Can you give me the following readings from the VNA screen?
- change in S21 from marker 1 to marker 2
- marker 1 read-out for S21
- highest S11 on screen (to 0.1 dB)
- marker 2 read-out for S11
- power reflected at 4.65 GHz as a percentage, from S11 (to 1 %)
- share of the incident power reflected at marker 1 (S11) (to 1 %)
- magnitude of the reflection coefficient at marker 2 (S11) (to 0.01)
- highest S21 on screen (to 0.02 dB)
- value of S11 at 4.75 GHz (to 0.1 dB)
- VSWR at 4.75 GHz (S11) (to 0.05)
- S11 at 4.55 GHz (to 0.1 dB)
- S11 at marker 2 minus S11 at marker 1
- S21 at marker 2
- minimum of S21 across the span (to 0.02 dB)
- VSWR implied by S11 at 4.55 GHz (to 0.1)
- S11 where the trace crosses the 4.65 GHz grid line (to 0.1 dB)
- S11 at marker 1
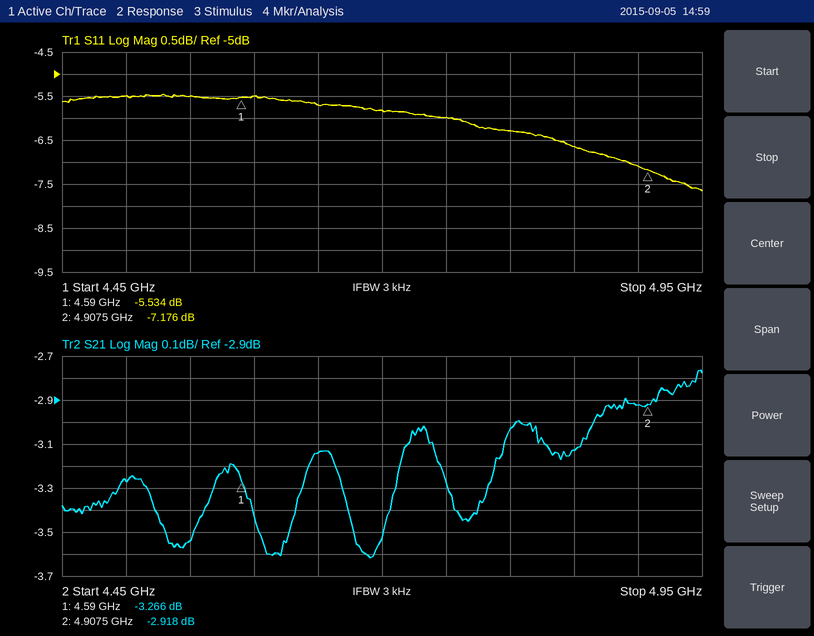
0.348 dB
-3.266 dB
-5.5 dB
-7.176 dB
27 %
28 %
0.44
-2.76 dB
-6.0 dB
3.00
-5.5 dB
-1.642 dB
-2.918 dB
-3.62 dB
3.3
-5.7 dB
-5.534 dB
